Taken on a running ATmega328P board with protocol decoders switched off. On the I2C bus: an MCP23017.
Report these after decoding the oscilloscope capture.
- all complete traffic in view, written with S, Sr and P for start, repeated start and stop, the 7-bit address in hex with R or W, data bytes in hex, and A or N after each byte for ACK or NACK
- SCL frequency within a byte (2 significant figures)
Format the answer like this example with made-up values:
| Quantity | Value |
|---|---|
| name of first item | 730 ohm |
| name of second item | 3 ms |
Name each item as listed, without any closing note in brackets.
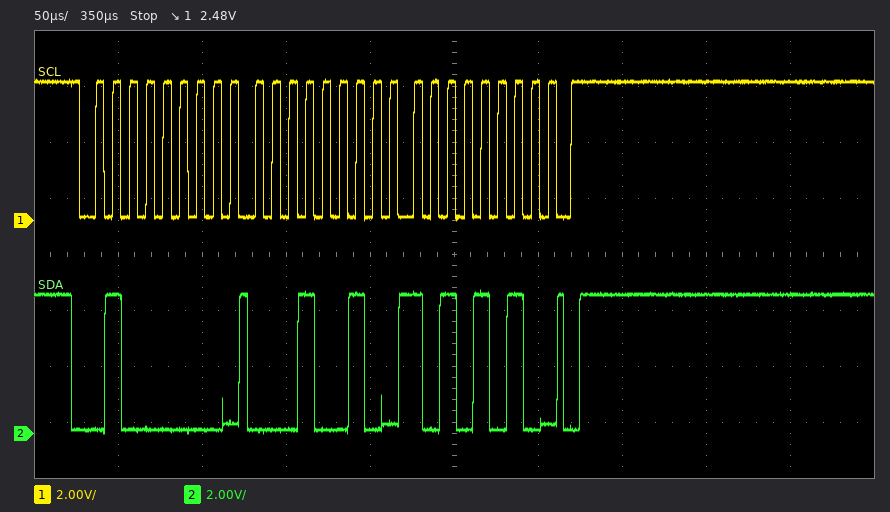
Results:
| Quantity | Value |
|---|---|
| all complete traffic in view, written with S, Sr and P for start, repeated start and stop, the 7-bit address in hex with R or W, data bytes in hex, and A or N after each byte for ACK or NACK | S 20W A 12 A AA A P |
| SCL frequency within a byte | 100 kHz |
